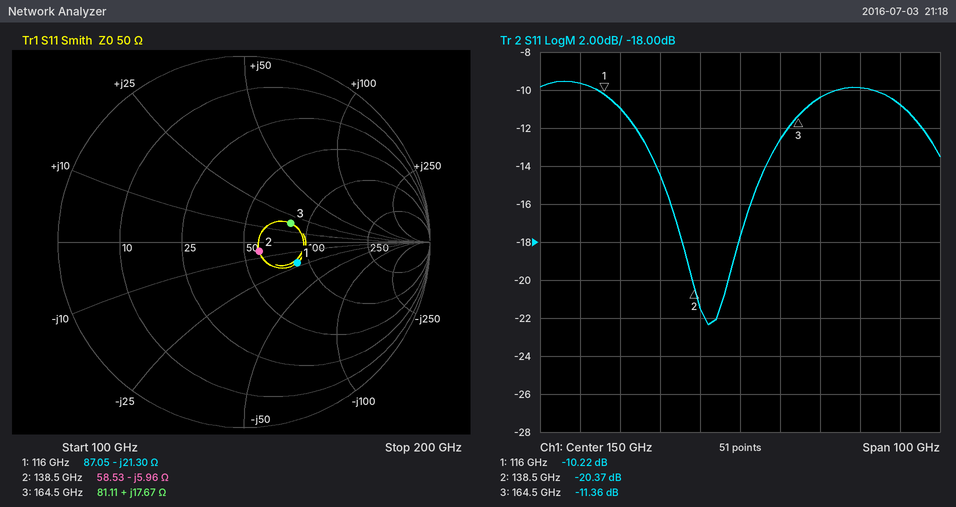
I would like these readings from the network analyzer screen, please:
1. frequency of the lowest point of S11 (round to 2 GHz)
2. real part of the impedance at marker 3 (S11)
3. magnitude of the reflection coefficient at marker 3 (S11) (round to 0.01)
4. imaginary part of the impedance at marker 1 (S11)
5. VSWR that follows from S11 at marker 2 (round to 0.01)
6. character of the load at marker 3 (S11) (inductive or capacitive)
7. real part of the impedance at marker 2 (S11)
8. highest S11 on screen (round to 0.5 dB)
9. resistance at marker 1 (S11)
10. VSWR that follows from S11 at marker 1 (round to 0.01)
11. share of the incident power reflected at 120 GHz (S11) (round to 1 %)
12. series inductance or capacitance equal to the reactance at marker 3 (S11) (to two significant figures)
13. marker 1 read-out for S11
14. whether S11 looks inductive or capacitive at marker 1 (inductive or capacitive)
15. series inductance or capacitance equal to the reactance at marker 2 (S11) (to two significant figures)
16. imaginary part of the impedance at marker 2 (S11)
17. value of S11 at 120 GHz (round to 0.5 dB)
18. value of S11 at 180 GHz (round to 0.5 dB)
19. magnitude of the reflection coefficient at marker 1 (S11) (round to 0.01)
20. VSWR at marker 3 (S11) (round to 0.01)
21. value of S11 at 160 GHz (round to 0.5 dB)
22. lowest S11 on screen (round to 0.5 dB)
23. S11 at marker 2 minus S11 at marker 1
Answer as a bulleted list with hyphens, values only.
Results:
- 142 GHz
- 81.11 Ω
- 0.27
- -21.30 Ω
- 1.21
- inductive
- 58.53 Ω
- -9.5 dB
- 87.05 Ω
- 1.89
- 8 %
- 17 pH
- -10.22 dB
- capacitive
- 190 fF
- -5.96 Ω
- -11.0 dB
- -10.0 dB
- 0.31
- 1.74
- -12.5 dB
- -22.5 dB
- -10.15 dB
